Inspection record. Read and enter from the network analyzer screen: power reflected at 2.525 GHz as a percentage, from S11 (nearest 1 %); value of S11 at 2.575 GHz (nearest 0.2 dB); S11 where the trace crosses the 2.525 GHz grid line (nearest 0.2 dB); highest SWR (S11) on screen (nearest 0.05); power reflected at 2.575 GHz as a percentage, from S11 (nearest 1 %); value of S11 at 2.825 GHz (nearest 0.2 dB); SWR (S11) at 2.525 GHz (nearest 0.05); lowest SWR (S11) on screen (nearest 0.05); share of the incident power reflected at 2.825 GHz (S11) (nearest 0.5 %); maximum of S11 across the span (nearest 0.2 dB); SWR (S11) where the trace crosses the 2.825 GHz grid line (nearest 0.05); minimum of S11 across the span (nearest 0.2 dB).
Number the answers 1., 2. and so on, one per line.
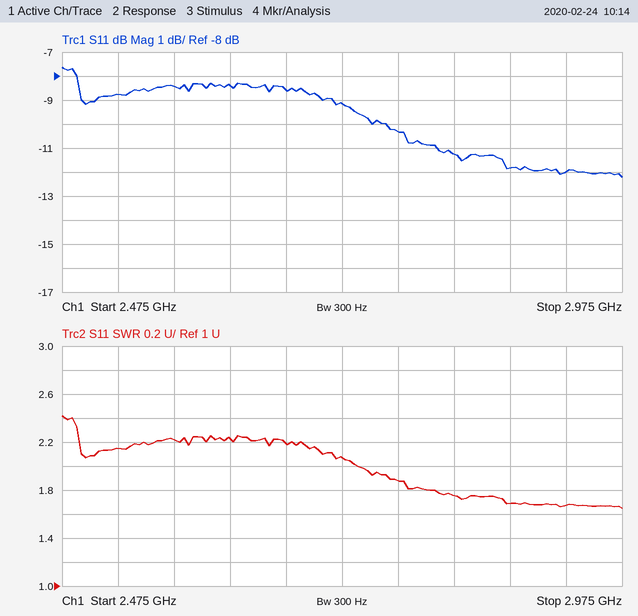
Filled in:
1. 13 %
2. -8.4 dB
3. -8.8 dB
4. 2.40
5. 14 %
6. -11.2 dB
7. 2.15
8. 1.65
9. 7.5 %
10. -7.6 dB
11. 1.75
12. -12.2 dB
